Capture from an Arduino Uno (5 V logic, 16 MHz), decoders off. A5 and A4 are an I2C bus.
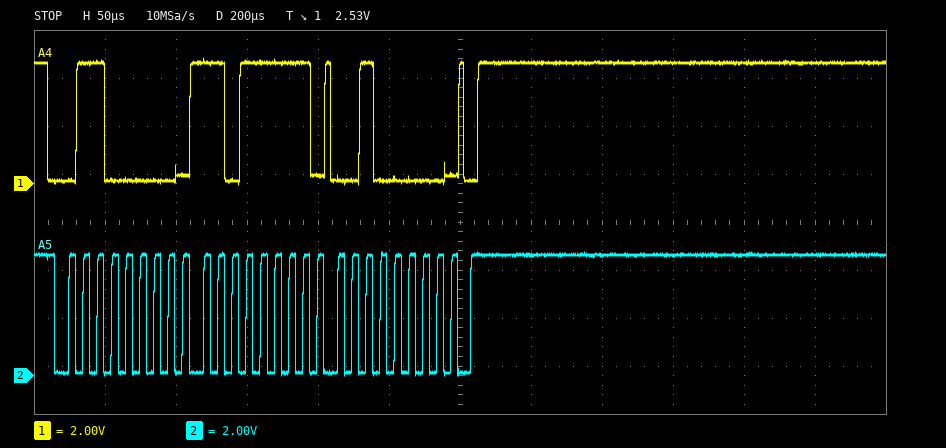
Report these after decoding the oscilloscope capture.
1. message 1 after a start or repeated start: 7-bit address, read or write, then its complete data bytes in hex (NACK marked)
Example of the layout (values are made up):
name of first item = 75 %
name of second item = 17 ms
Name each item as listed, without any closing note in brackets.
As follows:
message 1 after a start or repeated start: 7-bit address, read or write, then its complete data bytes in hex = 0x30 write: DF 20
